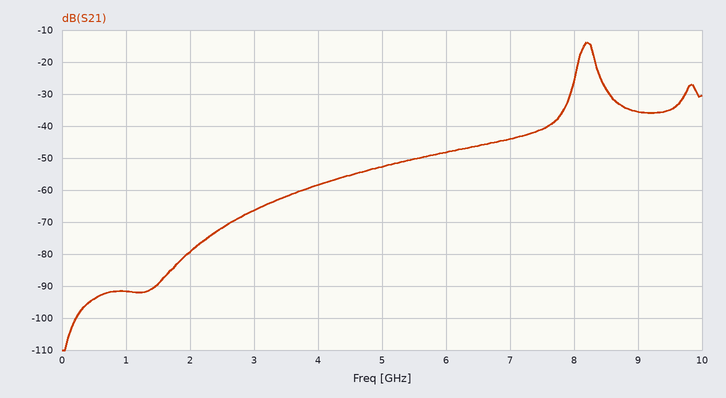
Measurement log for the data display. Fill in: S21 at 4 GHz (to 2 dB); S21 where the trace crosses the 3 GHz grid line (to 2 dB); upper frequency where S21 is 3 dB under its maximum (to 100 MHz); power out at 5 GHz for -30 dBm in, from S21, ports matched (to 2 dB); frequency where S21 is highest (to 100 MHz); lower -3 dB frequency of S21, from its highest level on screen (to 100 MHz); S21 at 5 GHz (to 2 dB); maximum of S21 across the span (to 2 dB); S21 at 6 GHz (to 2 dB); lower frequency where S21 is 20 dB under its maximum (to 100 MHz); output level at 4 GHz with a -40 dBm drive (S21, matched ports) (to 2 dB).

-58 dB
-66 dB
8.3 GHz
-82 dBm
8.2 GHz
8.1 GHz
-52 dB
-14 dB
-48 dB
7.9 GHz
-98 dBm
